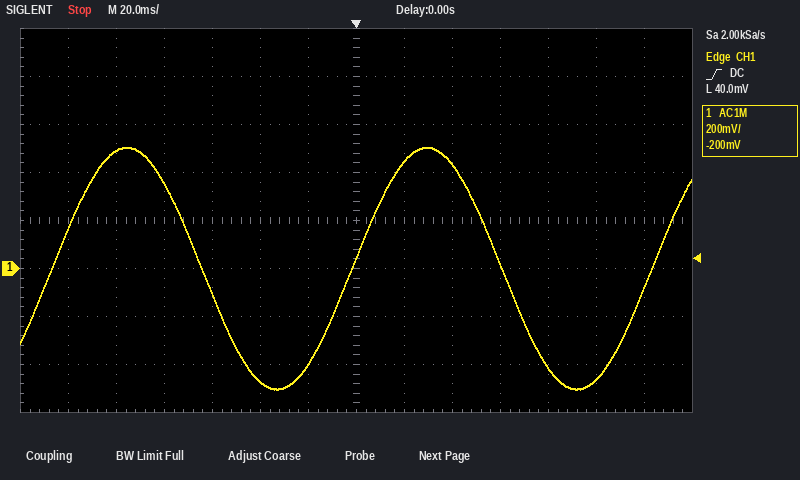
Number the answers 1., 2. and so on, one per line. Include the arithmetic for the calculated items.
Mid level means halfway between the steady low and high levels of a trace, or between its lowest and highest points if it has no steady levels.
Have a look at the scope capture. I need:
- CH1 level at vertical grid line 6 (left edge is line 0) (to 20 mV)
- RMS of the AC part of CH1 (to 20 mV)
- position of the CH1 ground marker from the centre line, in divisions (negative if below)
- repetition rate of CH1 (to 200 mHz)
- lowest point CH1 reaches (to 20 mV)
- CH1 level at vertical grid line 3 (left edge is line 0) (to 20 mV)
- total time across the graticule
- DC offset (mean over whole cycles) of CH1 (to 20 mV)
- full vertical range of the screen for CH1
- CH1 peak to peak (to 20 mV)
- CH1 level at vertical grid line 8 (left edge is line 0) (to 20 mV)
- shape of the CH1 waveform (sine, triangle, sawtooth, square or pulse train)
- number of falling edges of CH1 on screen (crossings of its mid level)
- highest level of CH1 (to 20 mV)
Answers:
1. -400 mV
2. 1.00 V / (2√2) ≈ 354 mV, so 360 mV to the nearest 20 mV
3. -1.0 div
4. 8.0 Hz
5. -500 mV
6. 360 mV
7. 280 ms
8. (500 mV + (-500 mV)) / 2 ≈ 0 mV
9. 1.6 V
10. 500 mV − (-500 mV) = 1.00 V
11. 440 mV
12. sine
13. 2
14. 500 mV
